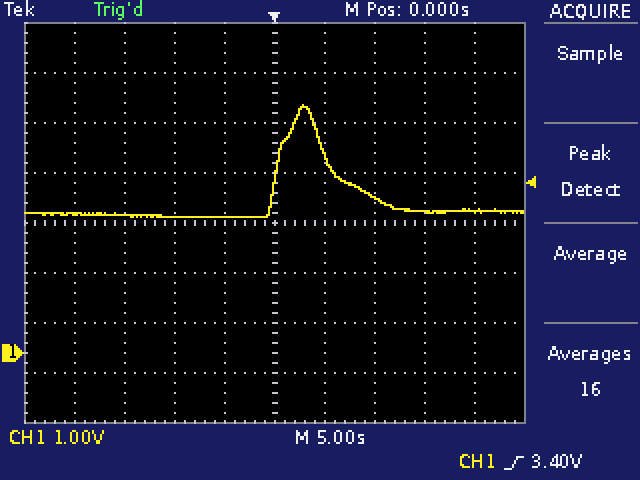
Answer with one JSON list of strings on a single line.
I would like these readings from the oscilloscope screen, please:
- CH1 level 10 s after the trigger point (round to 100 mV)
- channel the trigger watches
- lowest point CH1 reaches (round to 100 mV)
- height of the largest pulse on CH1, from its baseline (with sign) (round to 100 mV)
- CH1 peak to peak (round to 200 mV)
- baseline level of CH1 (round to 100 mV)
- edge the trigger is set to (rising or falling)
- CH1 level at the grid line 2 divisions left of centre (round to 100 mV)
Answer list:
["3.1 V", "CH1", "2.7 V", "+2.2 V", "2.2 V", "2.8 V", "rising", "2.7 V"]
